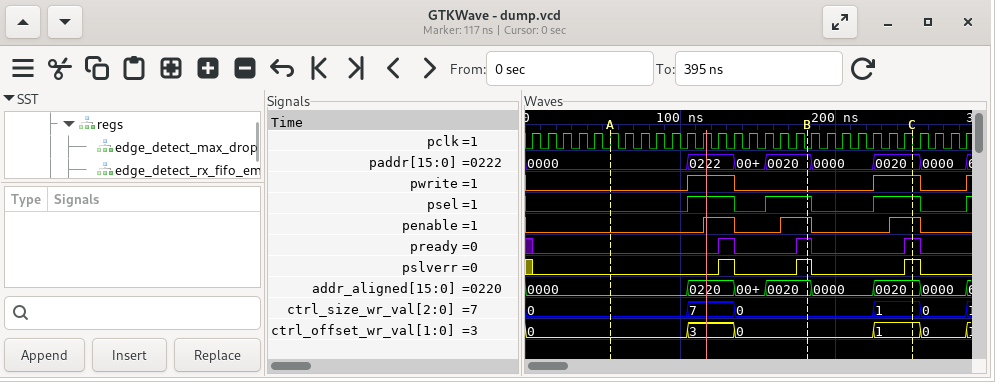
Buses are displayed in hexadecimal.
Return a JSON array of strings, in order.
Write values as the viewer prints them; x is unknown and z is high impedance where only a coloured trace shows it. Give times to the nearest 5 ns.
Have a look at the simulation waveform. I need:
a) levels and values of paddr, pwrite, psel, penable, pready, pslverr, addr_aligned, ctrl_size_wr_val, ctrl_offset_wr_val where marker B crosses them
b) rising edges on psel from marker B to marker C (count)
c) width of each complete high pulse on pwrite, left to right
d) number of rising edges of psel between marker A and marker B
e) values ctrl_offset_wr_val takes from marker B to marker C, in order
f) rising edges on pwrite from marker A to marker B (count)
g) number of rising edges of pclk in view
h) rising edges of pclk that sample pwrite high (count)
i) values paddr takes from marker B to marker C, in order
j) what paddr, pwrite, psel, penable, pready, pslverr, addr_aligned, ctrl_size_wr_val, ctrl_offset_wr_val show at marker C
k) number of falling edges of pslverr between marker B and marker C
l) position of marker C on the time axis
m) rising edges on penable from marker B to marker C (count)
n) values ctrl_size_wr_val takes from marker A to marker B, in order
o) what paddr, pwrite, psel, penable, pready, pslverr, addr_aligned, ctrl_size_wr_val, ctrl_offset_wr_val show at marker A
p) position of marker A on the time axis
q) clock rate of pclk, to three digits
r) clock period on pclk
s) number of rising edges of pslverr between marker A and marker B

["paddr=0020, pwrite=0, psel=1, penable=1, pready=1, pslverr=1, addr_aligned=0020, ctrl_size_wr_val=0, ctrl_offset_wr_val=0", "1", "30 ns, 30 ns", "2", "0, 1", "1", "29", "6", "0020, 0000, 0020", "paddr=0020, pwrite=1, psel=1, penable=1, pready=1, pslverr=1, addr_aligned=0020, ctrl_size_wr_val=1, ctrl_offset_wr_val=1", "1", "250 ns", "1", "0, 7, 0", "paddr=0000, pwrite=0, psel=0, penable=0, pready=0, pslverr=0, addr_aligned=0000, ctrl_size_wr_val=0, ctrl_offset_wr_val=0", "55 ns", "100 MHz", "10 ns", "2"]
